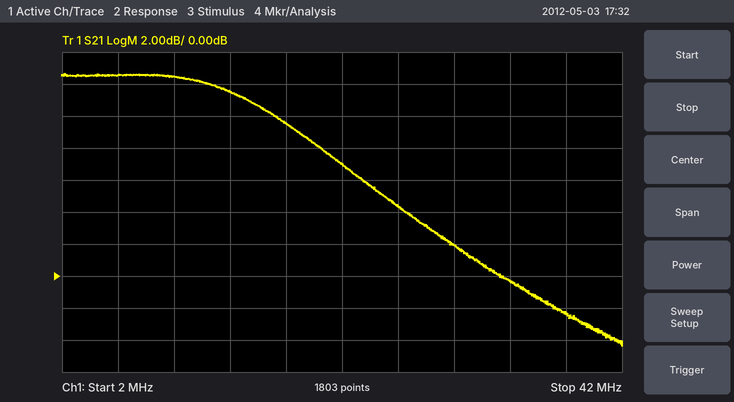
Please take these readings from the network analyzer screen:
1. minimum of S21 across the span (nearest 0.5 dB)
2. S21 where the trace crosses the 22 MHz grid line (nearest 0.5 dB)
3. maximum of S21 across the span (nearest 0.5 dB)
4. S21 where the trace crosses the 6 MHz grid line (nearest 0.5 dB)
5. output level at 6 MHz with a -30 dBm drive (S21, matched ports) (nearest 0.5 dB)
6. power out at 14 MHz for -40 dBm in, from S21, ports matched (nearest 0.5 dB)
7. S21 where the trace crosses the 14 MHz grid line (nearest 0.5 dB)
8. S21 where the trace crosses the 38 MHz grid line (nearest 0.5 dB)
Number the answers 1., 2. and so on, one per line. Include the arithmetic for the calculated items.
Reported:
1. -4.5 dB
2. 7.0 dB
3. 12.5 dB
4. 12.5 dB
5. -30 dBm + (12.5 dB) = -17.5 dBm
6. -40 dBm + (11.5 dB) = -28.5 dBm
7. 11.5 dB
8. -2.5 dB
